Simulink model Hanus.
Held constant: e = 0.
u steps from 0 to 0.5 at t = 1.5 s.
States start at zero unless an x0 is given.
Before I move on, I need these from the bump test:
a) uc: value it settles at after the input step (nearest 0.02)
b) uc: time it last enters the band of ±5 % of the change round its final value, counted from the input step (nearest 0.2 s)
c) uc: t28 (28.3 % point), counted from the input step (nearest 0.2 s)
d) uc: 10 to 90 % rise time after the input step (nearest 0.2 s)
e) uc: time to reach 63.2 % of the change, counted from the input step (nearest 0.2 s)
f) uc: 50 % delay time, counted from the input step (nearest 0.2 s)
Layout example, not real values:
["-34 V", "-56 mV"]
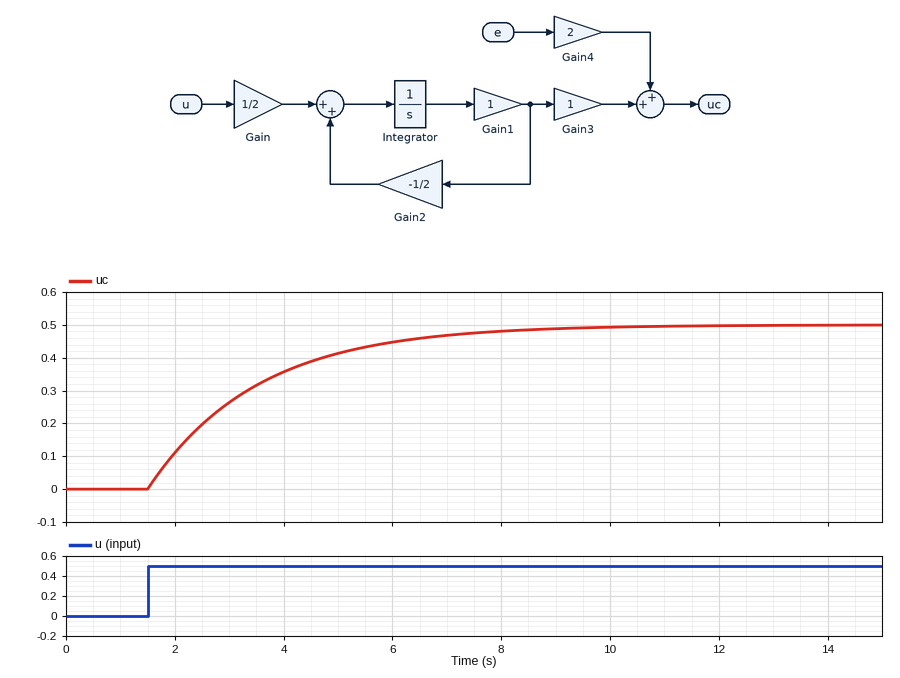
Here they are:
["0.50", "6.0 s", "0.6 s", "4.4 s", "2.0 s", "1.4 s"]
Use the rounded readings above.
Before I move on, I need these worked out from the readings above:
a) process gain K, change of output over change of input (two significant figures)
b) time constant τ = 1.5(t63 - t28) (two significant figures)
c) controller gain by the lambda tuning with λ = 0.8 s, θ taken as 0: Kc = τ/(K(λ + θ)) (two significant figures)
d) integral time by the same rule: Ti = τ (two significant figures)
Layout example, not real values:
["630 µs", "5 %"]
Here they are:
["1.0", "2.1 s", "2.6", "2.1 s"]
